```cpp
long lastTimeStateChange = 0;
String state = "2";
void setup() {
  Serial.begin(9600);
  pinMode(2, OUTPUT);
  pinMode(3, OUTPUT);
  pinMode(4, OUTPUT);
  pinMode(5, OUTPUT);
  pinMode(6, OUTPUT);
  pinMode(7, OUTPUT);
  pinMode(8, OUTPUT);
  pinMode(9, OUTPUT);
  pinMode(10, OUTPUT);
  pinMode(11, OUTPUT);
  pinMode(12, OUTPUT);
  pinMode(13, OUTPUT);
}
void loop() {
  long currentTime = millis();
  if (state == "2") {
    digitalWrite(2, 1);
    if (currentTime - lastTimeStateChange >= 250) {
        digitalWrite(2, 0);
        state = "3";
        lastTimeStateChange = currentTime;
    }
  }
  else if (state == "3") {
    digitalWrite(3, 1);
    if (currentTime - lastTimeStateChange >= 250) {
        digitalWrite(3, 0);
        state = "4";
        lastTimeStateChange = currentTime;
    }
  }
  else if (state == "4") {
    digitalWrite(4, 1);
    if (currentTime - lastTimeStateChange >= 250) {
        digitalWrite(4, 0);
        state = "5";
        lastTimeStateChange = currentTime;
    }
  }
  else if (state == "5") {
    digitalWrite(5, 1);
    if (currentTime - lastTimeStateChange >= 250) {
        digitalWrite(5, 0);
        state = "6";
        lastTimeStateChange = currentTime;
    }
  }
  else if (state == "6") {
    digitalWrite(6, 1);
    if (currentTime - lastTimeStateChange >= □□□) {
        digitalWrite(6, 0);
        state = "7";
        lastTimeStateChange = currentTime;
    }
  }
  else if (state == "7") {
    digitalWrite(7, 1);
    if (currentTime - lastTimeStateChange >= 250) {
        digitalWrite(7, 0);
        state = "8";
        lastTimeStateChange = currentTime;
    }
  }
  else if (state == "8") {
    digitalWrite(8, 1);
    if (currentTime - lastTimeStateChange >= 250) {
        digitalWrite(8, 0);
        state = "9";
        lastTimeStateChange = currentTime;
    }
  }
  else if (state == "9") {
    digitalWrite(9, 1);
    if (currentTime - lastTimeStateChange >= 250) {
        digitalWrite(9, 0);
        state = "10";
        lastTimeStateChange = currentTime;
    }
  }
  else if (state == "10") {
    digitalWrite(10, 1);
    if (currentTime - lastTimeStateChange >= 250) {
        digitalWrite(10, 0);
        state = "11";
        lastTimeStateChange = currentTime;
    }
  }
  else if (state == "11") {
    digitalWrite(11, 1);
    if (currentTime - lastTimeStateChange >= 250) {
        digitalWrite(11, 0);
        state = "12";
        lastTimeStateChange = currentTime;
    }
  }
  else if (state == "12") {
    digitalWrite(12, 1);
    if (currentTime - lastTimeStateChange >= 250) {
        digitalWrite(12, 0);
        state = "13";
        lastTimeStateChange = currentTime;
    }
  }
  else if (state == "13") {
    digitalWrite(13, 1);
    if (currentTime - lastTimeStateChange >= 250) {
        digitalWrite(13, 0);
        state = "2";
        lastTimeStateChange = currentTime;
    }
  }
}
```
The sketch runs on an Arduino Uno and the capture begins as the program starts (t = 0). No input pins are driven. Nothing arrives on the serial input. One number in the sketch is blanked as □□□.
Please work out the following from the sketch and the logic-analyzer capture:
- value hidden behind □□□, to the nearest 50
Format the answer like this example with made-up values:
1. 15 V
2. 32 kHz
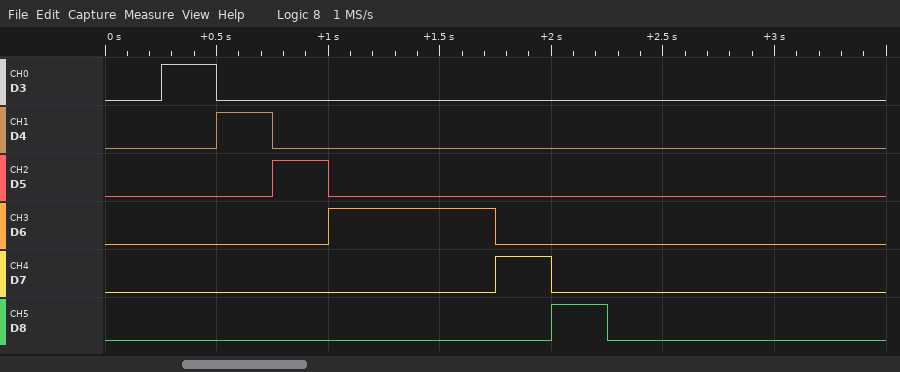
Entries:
1. 750
